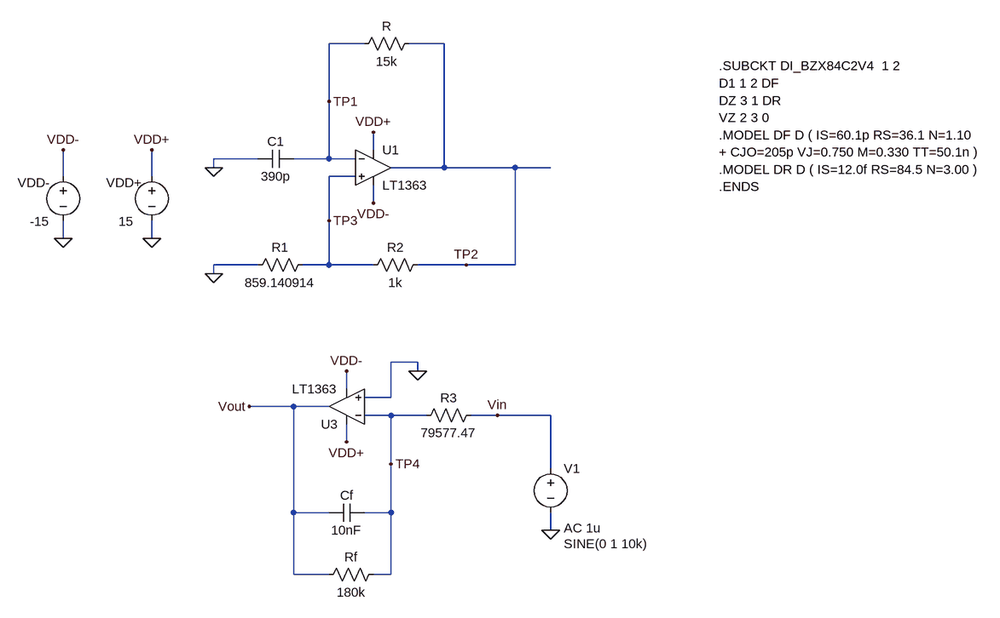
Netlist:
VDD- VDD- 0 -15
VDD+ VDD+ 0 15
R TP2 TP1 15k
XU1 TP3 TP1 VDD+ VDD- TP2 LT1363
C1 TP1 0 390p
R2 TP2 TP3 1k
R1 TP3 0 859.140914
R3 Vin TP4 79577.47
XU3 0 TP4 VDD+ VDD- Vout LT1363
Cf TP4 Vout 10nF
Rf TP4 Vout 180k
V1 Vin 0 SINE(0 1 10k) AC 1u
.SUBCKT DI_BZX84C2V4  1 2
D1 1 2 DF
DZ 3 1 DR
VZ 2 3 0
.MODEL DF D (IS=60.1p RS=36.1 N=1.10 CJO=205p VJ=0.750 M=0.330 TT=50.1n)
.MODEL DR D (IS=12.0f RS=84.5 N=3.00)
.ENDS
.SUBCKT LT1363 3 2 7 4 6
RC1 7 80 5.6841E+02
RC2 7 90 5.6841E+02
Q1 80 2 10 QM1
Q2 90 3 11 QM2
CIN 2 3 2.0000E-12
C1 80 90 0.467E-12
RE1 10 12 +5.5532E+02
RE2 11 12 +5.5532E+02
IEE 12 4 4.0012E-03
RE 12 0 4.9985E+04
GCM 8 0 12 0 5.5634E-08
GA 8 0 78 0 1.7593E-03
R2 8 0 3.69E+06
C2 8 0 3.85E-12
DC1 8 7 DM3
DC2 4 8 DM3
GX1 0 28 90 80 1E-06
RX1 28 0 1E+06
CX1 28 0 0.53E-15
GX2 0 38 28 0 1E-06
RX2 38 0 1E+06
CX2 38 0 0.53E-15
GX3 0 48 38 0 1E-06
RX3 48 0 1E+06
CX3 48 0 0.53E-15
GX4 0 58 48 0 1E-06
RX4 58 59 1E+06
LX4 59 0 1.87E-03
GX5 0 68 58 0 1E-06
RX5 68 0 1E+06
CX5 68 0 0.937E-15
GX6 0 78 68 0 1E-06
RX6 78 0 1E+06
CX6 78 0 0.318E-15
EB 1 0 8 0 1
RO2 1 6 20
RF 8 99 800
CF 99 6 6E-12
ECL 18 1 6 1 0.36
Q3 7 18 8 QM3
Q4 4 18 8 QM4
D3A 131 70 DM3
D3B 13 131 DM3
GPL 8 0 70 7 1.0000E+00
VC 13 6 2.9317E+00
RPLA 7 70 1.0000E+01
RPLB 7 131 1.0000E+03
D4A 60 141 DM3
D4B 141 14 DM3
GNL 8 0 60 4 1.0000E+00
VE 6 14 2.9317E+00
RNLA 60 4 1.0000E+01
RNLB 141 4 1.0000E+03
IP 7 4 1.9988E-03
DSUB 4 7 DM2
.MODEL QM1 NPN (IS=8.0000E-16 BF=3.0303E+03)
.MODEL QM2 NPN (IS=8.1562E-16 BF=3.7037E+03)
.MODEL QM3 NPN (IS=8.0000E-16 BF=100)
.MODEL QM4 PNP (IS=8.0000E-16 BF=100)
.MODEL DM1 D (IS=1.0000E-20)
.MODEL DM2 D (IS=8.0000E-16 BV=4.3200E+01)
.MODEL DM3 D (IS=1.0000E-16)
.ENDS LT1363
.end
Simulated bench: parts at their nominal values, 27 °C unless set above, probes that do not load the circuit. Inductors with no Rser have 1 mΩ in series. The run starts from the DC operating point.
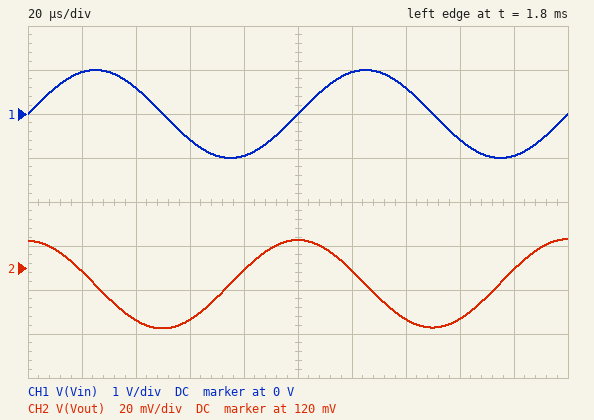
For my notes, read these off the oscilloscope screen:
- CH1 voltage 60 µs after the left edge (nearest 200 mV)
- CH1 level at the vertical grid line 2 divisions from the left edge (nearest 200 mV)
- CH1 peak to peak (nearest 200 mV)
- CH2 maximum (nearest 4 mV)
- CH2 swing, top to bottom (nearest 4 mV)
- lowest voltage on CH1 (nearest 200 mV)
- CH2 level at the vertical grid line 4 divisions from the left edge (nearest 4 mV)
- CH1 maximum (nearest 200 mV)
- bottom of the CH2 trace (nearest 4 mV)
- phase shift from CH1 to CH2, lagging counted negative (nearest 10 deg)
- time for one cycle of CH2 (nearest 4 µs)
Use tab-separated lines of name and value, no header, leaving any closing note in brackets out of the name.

CH1 voltage 60 µs after the left edge	-600 mV
CH1 level at the vertical grid line 2 divisions from the left edge	600 mV
CH1 peak to peak	2.0 V
CH2 maximum	132 mV
CH2 swing, top to bottom	40 mV
lowest voltage on CH1	-1.0 V
CH2 level at the vertical grid line 4 divisions from the left edge	120 mV
CH1 maximum	1.0 V
bottom of the CH2 trace	92 mV
phase shift from CH1 to CH2, lagging counted negative	90 deg
time for one cycle of CH2	100 µs
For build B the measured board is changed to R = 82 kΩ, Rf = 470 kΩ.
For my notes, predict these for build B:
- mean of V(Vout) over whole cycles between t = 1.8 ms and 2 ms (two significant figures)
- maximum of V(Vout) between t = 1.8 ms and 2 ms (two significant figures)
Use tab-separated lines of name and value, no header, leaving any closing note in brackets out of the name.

mean of V(Vout) over whole cycles between t = 1.8 ms and 2 ms	300 mV
maximum of V(Vout) between t = 1.8 ms and 2 ms	320 mV
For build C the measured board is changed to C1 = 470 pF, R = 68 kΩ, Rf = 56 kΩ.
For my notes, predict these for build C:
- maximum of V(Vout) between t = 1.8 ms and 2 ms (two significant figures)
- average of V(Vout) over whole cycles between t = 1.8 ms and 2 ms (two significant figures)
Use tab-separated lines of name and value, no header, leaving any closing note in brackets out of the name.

maximum of V(Vout) between t = 1.8 ms and 2 ms	57 mV
average of V(Vout) over whole cycles between t = 1.8 ms and 2 ms	37 mV
